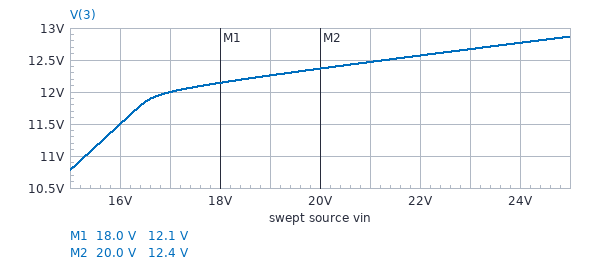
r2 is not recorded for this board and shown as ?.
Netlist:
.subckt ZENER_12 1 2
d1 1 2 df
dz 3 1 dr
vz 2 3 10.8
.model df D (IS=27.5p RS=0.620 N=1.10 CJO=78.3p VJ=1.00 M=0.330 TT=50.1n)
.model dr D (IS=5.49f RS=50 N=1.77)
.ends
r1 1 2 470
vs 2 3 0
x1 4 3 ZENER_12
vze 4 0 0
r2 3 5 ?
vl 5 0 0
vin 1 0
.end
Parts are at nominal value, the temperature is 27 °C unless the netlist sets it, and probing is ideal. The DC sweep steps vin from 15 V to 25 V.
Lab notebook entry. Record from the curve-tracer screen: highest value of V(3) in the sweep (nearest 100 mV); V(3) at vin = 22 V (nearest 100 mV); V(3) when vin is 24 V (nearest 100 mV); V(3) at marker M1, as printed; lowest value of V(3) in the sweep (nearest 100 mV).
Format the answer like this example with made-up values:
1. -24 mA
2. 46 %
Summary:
1. 12.9 V
2. 12.6 V
3. 12.8 V
4. 12.1 V
5. 10.8 V
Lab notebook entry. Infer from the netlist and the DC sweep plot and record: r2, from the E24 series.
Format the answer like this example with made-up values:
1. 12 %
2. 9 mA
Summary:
1. 1.2 kΩ
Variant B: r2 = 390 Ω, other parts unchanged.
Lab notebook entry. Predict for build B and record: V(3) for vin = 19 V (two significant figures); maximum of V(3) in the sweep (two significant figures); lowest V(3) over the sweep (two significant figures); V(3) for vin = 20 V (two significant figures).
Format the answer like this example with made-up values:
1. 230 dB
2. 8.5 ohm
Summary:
1. 8.6 V
2. 11 V
3. 6.8 V
4. 9.1 V
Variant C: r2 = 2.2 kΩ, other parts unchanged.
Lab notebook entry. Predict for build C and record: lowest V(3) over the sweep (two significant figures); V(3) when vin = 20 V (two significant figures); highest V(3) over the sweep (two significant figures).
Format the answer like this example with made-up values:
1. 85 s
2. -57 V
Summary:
1. 12 V
2. 13 V
3. 13 V
